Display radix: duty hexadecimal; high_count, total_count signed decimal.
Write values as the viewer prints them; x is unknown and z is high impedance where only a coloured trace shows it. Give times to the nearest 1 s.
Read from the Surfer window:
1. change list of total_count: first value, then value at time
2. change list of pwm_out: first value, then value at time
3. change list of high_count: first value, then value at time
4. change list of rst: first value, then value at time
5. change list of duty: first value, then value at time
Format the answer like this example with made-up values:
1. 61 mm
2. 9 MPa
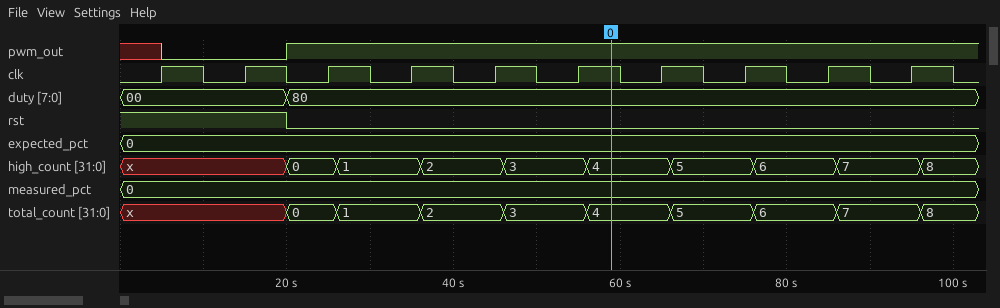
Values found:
1. x, 0 at 20 s, 1 at 26 s, 2 at 36 s, 3 at 46 s, 4 at 56 s, 5 at 66 s, 6 at 76 s, 7 at 86 s, 8 at 96 s
2. x, 0 at 5 s, 1 at 20 s
3. x, 0 at 20 s, 1 at 26 s, 2 at 36 s, 3 at 46 s, 4 at 56 s, 5 at 66 s, 6 at 76 s, 7 at 86 s, 8 at 96 s
4. 1, 0 at 20 s
5. 00, 80 at 20 s
